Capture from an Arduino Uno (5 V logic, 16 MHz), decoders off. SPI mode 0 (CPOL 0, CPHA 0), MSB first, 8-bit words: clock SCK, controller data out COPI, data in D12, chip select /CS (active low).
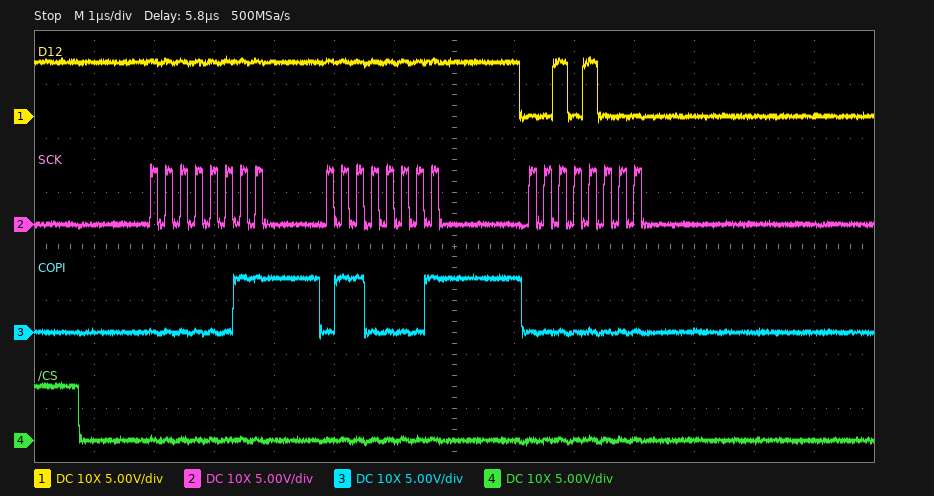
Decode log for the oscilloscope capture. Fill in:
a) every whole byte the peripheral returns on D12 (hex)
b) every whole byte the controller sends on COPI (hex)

FF FF 28
03 61 00
